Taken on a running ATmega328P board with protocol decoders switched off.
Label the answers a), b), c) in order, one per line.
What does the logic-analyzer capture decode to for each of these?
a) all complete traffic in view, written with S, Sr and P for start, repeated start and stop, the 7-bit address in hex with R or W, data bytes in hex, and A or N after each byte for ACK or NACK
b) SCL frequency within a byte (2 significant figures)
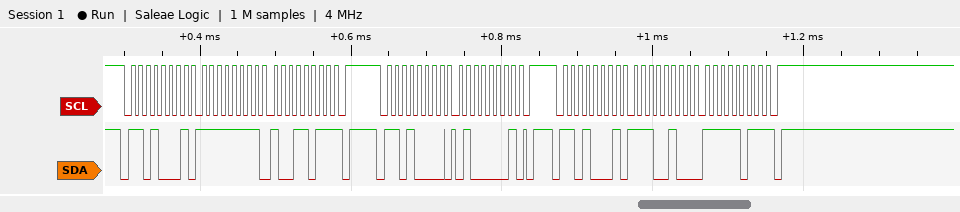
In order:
a) S 68R A FF A 9B N P S 68W A 41 A P S 68R A E4 A FB N P
b) 100 kHz
